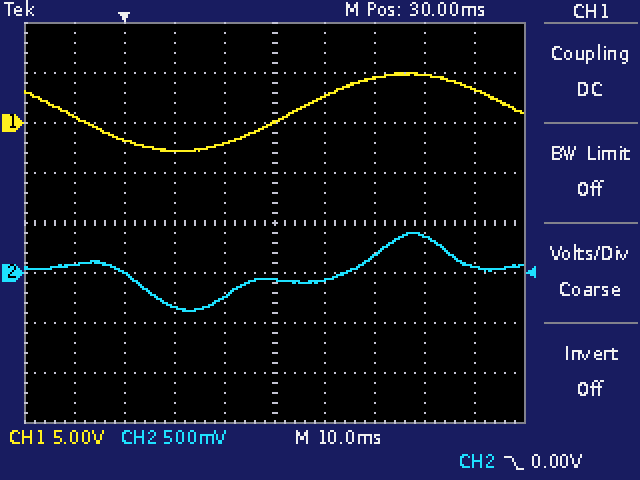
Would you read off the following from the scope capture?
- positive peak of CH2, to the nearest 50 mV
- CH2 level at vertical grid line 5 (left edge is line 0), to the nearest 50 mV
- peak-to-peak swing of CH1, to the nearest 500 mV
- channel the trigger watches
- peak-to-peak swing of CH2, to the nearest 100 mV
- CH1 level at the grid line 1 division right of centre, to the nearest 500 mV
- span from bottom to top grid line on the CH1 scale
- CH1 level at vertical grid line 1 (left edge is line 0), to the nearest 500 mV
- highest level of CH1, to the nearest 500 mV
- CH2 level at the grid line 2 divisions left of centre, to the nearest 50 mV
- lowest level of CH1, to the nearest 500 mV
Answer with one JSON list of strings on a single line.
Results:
["400 mV", "-50 mV", "8.0 V", "CH2", "800 mV", "2.5 V", "40 V", "500 mV", "5.0 V", "-350 mV", "-3.0 V"]
